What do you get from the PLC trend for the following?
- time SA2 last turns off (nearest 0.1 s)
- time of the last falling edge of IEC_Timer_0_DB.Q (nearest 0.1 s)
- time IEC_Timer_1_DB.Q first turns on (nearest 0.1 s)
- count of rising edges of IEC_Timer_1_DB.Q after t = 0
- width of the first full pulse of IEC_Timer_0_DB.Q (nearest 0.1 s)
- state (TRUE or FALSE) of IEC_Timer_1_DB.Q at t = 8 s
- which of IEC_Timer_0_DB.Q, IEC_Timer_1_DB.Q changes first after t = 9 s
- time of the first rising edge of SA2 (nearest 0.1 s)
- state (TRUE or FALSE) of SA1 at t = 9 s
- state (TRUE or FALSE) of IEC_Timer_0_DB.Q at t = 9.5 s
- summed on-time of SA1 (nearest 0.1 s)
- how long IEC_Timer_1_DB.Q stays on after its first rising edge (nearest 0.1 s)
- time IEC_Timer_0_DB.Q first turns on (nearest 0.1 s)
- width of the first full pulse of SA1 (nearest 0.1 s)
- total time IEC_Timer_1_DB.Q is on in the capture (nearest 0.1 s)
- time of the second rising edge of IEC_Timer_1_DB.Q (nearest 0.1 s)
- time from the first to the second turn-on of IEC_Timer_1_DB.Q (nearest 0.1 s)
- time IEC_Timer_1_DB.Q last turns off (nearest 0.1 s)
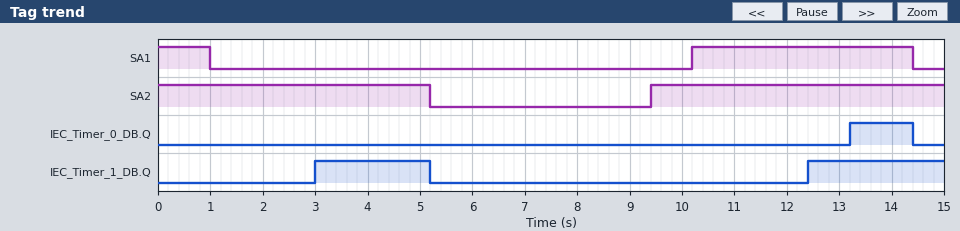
5.2 s
14.4 s
3.0 s
2
1.2 s
FALSE
IEC_Timer_1_DB.Q
9.4 s
FALSE
FALSE
5.2 s
2.2 s
13.2 s
4.2 s
4.8 s
12.4 s
9.4 s
5.2 s
